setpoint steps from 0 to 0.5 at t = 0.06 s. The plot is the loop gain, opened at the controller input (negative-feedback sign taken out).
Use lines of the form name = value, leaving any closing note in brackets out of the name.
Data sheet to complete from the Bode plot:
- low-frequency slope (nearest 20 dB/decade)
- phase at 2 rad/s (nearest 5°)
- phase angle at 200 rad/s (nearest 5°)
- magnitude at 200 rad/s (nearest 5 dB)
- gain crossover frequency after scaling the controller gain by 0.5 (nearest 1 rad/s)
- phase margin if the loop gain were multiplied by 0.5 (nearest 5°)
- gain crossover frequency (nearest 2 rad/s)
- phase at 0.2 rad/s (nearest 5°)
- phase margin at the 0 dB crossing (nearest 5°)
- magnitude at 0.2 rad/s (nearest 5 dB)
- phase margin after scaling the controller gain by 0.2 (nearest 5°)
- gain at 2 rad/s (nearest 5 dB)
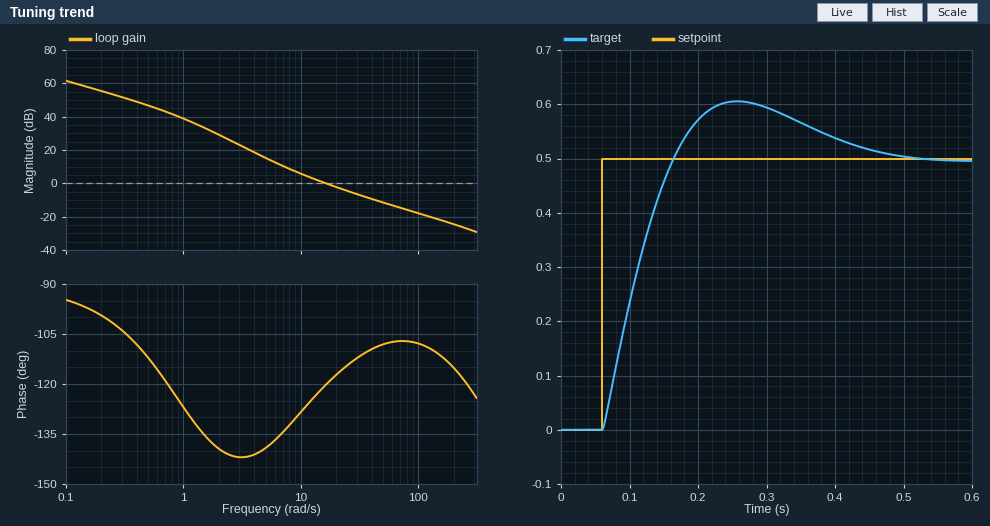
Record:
low-frequency slope = -20 dB/decade
phase at 2 rad/s = -140°
phase angle at 200 rad/s = -115°
magnitude at 200 rad/s = -25 dB
gain crossover frequency after scaling the controller gain by 0.5 = 10 rad/s
phase margin if the loop gain were multiplied by 0.5 = 50°
gain crossover frequency = 16 rad/s
phase at 0.2 rad/s = -100°
phase margin at the 0 dB crossing = 60°
magnitude at 0.2 rad/s = 55 dB
phase margin after scaling the controller gain by 0.2 = 40°
gain at 2 rad/s = 30 dB
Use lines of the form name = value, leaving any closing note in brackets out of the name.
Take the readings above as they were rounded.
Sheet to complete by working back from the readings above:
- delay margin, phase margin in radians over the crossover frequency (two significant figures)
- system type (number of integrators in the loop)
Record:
delay margin, phase margin in radians over the crossover frequency = 0.065 s
system type = 1
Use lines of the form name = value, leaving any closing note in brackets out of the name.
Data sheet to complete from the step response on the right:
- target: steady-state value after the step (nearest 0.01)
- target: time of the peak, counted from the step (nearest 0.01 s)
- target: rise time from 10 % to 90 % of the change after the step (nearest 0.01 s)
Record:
target: steady-state value after the step = 0.50
target: time of the peak, counted from the step = 0.20 s
target: rise time from 10 % to 90 % of the change after the step = 0.08 s
